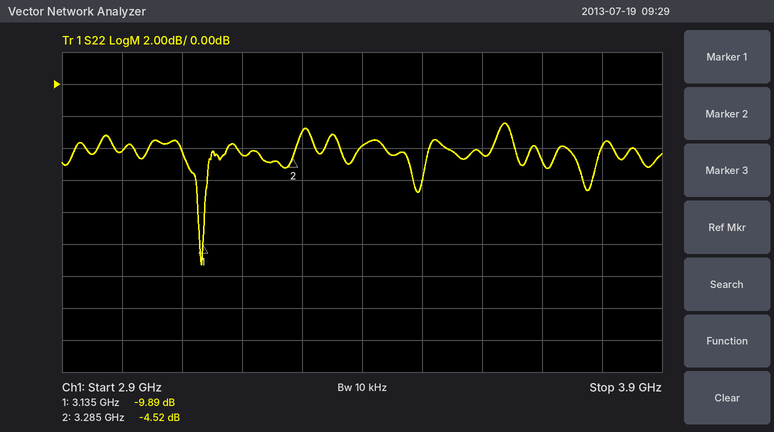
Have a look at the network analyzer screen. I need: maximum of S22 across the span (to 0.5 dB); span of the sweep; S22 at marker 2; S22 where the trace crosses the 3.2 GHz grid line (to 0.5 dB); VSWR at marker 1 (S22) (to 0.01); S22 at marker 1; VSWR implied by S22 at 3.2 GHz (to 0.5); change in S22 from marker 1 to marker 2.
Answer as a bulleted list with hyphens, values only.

- -2.5 dB
- 1 GHz
- -4.52 dB
- -4.5 dB
- 1.94
- -9.89 dB
- 4.0
- 5.37 dB
